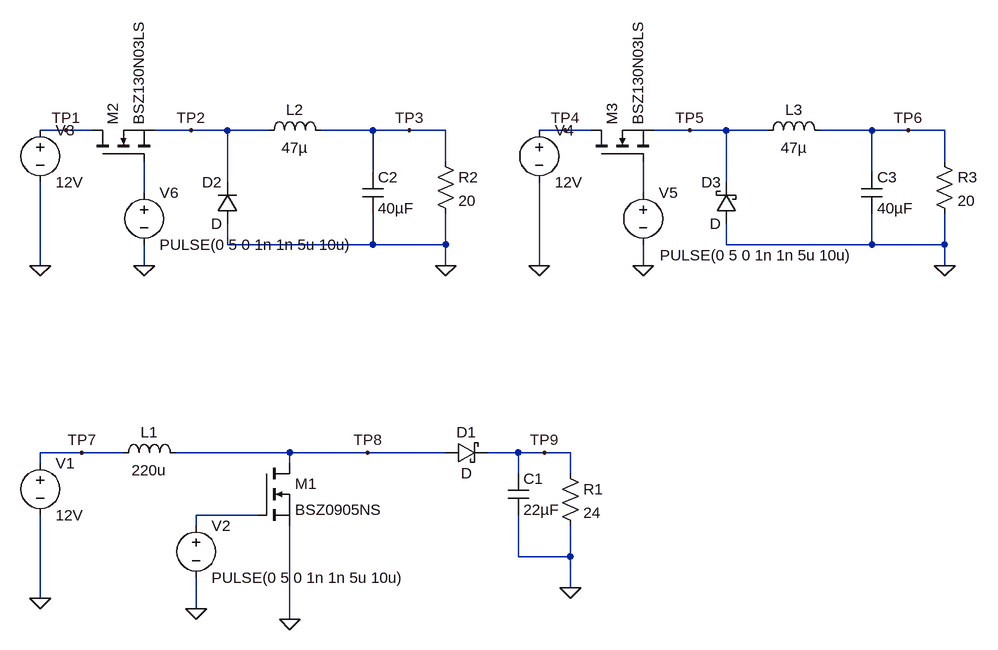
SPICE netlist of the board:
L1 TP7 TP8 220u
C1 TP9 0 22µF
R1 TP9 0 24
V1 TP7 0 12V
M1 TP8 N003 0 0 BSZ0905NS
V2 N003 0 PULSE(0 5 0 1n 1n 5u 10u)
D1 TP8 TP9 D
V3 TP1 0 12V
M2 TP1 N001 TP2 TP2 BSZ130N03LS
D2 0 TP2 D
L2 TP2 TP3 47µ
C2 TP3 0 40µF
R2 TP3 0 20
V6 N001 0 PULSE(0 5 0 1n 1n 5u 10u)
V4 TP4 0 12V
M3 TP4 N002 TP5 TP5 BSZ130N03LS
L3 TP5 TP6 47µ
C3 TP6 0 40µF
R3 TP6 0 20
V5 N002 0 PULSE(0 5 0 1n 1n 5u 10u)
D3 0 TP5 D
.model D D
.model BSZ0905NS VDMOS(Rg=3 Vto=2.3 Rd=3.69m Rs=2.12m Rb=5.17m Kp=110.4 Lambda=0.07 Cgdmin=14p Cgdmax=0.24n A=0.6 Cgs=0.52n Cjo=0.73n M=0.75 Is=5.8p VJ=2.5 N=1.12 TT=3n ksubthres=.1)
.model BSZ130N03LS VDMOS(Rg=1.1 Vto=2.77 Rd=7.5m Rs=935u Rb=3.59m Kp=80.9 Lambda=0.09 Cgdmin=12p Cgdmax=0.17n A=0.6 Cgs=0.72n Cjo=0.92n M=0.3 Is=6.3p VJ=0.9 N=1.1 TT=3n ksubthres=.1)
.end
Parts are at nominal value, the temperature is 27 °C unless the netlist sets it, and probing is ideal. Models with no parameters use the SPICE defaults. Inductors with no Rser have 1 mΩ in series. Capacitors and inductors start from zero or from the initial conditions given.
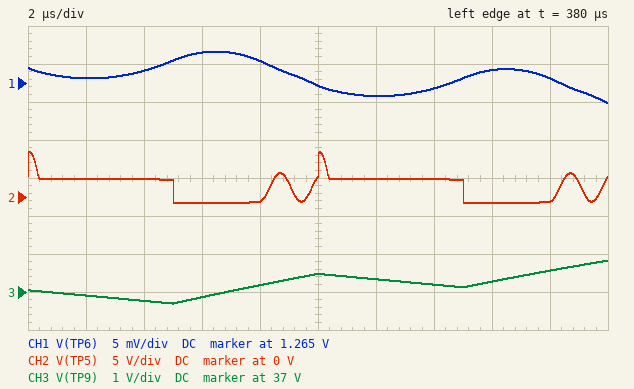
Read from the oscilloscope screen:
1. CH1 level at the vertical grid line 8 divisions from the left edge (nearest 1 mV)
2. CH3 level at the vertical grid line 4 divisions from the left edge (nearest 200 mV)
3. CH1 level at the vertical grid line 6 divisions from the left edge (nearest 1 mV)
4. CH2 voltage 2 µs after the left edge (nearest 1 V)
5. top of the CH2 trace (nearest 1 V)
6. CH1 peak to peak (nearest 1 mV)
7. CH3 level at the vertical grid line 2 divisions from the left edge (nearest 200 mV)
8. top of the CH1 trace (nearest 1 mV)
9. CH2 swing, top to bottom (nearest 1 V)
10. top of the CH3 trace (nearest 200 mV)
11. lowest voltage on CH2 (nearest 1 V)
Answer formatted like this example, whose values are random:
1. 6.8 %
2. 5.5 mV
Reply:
1. 1.267 V
2. 37.2 V
3. 1.263 V
4. 2 V
5. 6 V
6. 7 mV
7. 36.8 V
8. 1.269 V
9. 7 V
10. 37.8 V
11. -1 V
